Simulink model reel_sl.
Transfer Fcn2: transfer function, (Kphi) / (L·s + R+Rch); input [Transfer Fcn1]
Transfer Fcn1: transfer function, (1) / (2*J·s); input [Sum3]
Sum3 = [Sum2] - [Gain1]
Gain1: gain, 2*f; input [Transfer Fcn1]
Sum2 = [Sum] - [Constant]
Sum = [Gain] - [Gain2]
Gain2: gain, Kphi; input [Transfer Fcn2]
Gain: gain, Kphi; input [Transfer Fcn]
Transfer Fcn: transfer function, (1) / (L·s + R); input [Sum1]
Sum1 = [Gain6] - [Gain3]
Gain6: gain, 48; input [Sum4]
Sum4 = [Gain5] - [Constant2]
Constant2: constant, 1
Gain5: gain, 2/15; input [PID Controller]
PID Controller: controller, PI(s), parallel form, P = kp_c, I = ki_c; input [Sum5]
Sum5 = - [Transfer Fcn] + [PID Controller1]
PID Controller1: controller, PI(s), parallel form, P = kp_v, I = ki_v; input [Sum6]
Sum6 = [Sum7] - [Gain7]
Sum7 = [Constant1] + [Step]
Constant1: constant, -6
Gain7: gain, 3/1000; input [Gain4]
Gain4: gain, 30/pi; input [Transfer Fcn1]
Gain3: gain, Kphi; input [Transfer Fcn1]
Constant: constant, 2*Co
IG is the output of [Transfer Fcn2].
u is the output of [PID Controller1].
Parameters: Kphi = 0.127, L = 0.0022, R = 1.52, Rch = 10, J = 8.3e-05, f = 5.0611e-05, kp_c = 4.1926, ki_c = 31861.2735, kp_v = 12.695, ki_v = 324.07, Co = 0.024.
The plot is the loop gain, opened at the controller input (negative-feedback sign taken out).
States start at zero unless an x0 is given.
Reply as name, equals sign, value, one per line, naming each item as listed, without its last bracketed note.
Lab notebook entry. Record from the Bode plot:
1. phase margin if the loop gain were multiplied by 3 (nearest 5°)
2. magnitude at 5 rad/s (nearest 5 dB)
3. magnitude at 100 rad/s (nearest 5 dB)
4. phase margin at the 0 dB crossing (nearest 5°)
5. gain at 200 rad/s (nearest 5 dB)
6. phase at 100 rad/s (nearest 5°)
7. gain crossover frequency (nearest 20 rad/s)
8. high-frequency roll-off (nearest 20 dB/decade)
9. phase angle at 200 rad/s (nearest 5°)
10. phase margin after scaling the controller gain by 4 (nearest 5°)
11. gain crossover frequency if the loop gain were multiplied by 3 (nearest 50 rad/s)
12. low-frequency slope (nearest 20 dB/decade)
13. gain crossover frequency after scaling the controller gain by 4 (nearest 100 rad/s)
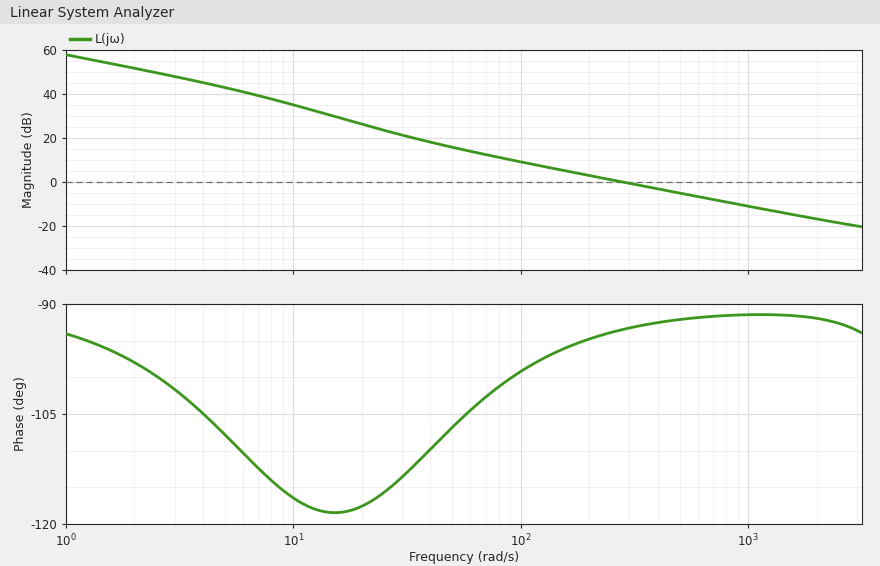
phase margin if the loop gain were multiplied by 3 = 90°
magnitude at 5 rad/s = 45 dB
magnitude at 100 rad/s = 10 dB
phase margin at the 0 dB crossing = 85°
gain at 200 rad/s = 5 dB
phase at 100 rad/s = -100°
gain crossover frequency = 280 rad/s
high-frequency roll-off = -20 dB/decade
phase angle at 200 rad/s = -95°
phase margin after scaling the controller gain by 4 = 90°
gain crossover frequency if the loop gain were multiplied by 3 = 850 rad/s
low-frequency slope = -20 dB/decade
gain crossover frequency after scaling the controller gain by 4 = 1100 rad/s
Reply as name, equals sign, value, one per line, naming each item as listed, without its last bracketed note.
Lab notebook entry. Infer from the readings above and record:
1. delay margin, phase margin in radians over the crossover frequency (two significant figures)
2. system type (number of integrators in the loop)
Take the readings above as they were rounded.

delay margin, phase margin in radians over the crossover frequency = 0.0053 s
system type = 1
